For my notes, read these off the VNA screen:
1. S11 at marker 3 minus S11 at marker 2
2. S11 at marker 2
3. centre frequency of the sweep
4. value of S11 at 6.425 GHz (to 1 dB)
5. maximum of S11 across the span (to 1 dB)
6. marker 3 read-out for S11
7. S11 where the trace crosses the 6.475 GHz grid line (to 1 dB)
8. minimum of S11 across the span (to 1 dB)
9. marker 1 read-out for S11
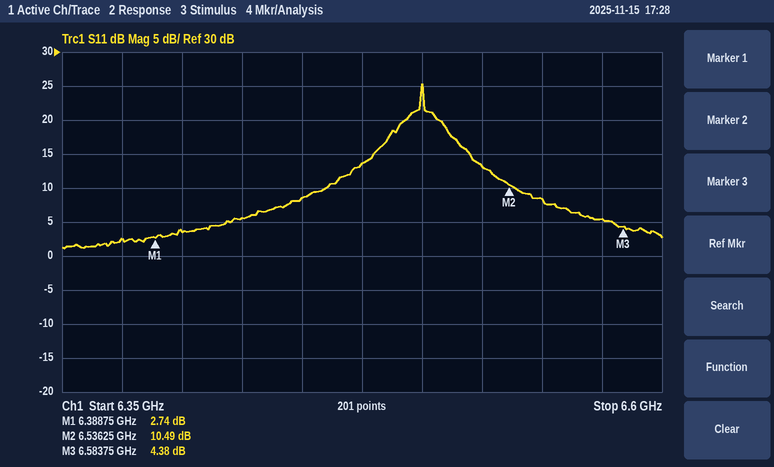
-6.11 dB
10.49 dB
6.475 GHz
6 dB
25 dB
4.38 dB
14 dB
1 dB
2.74 dB
